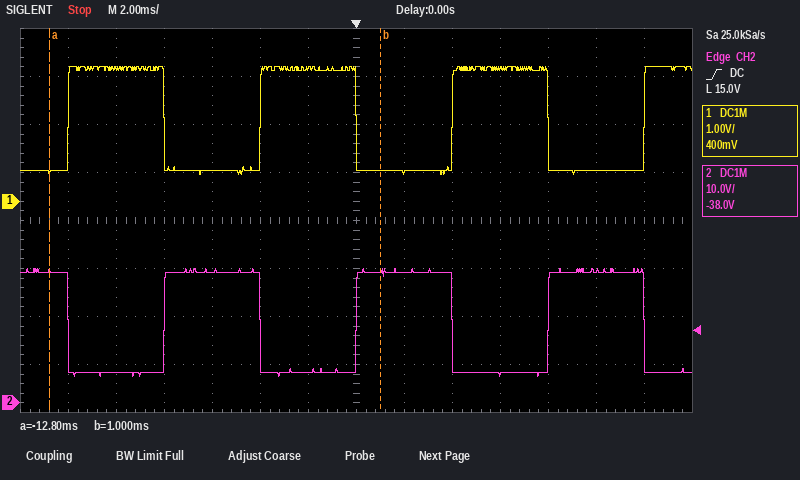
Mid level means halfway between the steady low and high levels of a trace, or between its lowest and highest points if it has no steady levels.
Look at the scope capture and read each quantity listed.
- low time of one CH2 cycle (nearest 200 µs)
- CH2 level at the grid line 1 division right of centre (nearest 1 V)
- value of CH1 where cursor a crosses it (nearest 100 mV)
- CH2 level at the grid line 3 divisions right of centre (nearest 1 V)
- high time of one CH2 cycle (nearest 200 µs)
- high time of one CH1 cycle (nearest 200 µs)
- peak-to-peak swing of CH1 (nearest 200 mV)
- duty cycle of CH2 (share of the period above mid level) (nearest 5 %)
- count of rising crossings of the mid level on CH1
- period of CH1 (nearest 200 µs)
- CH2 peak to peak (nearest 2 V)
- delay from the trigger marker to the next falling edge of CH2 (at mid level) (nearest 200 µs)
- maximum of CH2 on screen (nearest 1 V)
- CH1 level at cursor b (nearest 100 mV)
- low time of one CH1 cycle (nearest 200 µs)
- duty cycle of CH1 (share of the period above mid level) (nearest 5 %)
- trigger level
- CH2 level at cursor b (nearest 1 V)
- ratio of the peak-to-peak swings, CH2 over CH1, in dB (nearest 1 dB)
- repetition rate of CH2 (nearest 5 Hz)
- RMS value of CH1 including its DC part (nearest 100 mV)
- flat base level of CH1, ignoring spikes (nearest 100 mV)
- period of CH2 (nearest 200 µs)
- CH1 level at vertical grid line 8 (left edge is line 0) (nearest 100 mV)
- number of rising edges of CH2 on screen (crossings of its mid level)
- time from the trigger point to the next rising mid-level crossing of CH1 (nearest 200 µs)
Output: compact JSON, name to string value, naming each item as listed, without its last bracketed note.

{"low time of one CH2 cycle": "4.0 ms", "CH2 level at the grid line 1 division right of centre": "27 V", "value of CH1 where cursor a crosses it": "600 mV", "CH2 level at the grid line 3 divisions right of centre": "6 V", "high time of one CH2 cycle": "4.0 ms", "high time of one CH1 cycle": "4.0 ms", "peak-to-peak swing of CH1": "2.2 V", "duty cycle of CH2 (share of the period above mid level)": "50 %", "count of rising crossings of the mid level on CH1": "4", "period of CH1": "8.0 ms", "CH2 peak to peak": "22 V", "delay from the trigger marker to the next falling edge of CH2 (at mid level)": "4.0 ms", "maximum of CH2 on screen": "28 V", "CH1 level at cursor b": "600 mV", "low time of one CH1 cycle": "4.0 ms", "duty cycle of CH1 (share of the period above mid level)": "50 %", "trigger level": "15.0 V", "CH2 level at cursor b": "27 V", "ratio of the peak-to-peak swings, CH2 over CH1, in dB": "20 dB", "repetition rate of CH2": "125 Hz", "RMS value of CH1 including its DC part": "2.0 V", "flat base level of CH1, ignoring spikes": "600 mV", "period of CH2": "8.0 ms", "CH1 level at vertical grid line 8 (left edge is line 0)": "600 mV", "number of rising edges of CH2 on screen": "3", "time from the trigger point to the next rising mid-level crossing of CH1": "4.0 ms"}
